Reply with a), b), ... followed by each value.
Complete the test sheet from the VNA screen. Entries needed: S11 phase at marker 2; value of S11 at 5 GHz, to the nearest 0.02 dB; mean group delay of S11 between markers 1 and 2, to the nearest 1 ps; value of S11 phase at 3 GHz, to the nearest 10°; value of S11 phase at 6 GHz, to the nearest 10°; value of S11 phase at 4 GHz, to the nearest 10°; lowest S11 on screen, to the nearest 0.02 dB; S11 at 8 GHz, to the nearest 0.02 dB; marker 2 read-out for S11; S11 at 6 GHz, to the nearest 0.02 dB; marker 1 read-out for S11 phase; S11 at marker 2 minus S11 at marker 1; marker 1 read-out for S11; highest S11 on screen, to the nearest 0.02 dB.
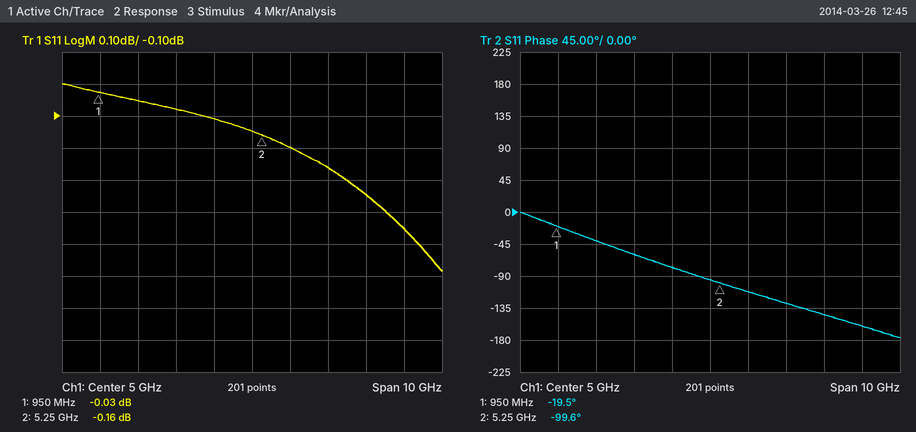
a) -99.6°
b) -0.14 dB
c) 52 ps
d) -60°
e) -110°
f) -80°
g) -0.58 dB
h) -0.34 dB
i) -0.16 dB
j) -0.20 dB
k) -19.5°
l) -0.13 dB
m) -0.03 dB
n) 0.00 dB
